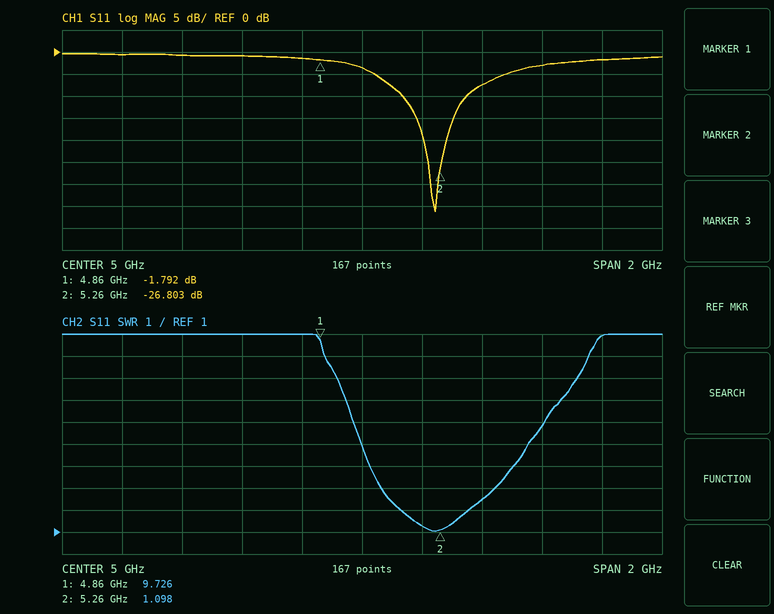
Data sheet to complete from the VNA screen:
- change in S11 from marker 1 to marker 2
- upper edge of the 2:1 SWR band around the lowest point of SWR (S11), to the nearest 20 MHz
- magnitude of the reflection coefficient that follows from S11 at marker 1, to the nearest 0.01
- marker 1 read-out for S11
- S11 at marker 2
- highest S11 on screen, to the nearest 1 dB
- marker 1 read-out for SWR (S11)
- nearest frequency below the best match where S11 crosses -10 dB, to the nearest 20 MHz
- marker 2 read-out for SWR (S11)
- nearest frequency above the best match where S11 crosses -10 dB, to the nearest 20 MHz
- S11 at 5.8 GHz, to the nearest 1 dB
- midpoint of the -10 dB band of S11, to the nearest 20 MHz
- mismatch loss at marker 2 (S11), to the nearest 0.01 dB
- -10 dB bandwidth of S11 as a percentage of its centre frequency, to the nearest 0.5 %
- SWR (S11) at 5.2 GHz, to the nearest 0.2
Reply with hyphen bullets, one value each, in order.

- -25.011 dB
- 5.36 GHz
- 0.81
- -1.792 dB
- -26.803 dB
- 0 dB
- 9.726
- 5.14 GHz
- 1.098
- 5.34 GHz
- -2 dB
- 5.24 GHz
- 0.01 dB
- 4.0 %
- 1.2
